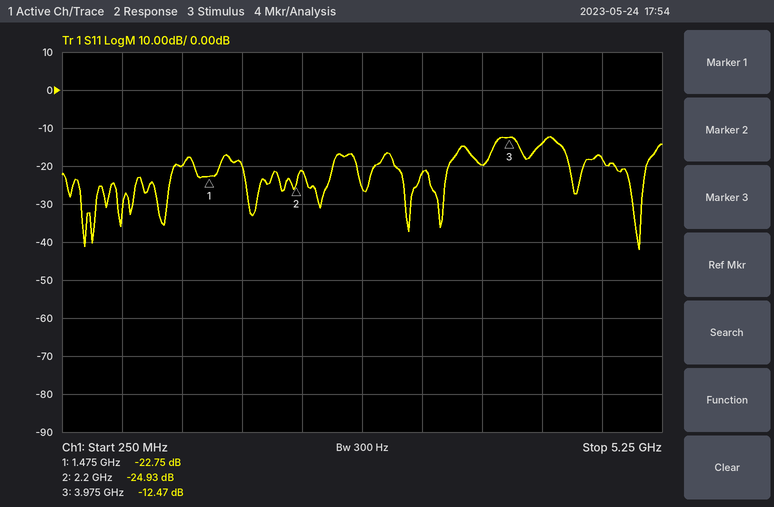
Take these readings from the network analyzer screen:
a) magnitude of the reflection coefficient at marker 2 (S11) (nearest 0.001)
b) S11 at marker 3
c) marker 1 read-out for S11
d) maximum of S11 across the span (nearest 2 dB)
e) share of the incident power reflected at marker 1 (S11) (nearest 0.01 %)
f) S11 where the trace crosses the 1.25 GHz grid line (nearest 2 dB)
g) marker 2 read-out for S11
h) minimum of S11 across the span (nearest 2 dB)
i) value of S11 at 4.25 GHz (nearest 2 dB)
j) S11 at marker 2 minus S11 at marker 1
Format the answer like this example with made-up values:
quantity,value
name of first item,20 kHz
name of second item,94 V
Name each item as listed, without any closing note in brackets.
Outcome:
quantity,value
magnitude of the reflection coefficient at marker 2 (S11),0.057
S11 at marker 3,-12.47 dB
marker 1 read-out for S11,-22.75 dB
maximum of S11 across the span,-12 dB
share of the incident power reflected at marker 1 (S11),0.53 %
S11 where the trace crosses the 1.25 GHz grid line,-20 dB
marker 2 read-out for S11,-24.93 dB
minimum of S11 across the span,-42 dB
value of S11 at 4.25 GHz,-14 dB
S11 at marker 2 minus S11 at marker 1,-2.18 dB
